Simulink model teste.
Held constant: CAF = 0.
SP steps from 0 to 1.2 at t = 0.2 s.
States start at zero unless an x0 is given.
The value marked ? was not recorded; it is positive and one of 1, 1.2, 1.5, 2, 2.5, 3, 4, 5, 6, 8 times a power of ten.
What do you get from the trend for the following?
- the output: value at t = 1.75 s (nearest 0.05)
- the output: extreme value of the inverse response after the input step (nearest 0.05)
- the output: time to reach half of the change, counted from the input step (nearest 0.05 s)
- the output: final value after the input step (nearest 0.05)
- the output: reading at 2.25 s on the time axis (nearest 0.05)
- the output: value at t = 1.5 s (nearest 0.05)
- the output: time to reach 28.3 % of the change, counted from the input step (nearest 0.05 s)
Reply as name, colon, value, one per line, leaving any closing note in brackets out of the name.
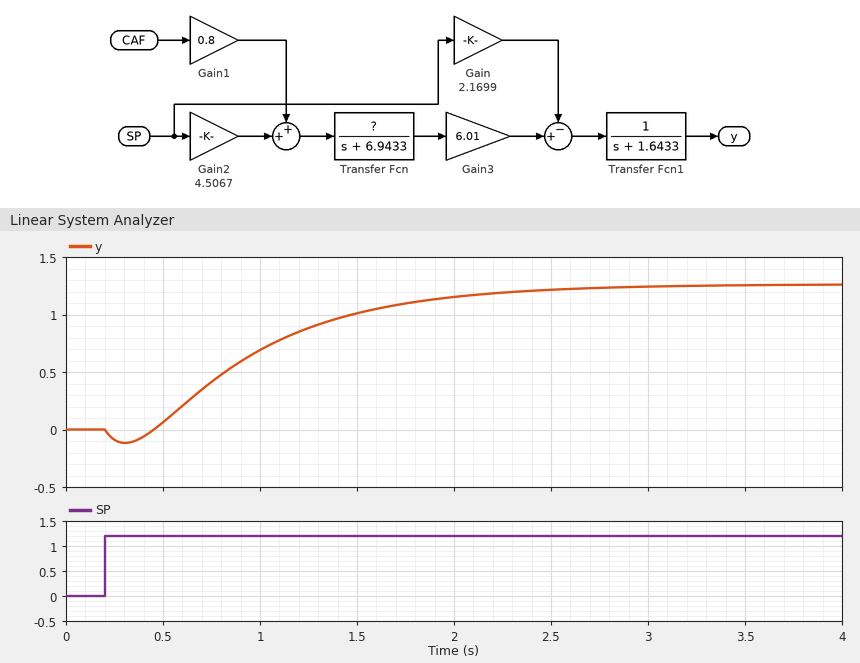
the output: value at t = 1.75 s: 1.10
the output: extreme value of the inverse response after the input step: -0.10
the output: time to reach half of the change, counted from the input step: 0.75 s
the output: final value after the input step: 1.25
the output: reading at 2.25 s on the time axis: 1.20
the output: value at t = 1.5 s: 1.00
the output: time to reach 28.3 % of the change, counted from the input step: 0.50 s
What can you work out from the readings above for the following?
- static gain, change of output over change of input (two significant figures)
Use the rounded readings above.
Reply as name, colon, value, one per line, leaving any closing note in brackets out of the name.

static gain, change of output over change of input: 1.0
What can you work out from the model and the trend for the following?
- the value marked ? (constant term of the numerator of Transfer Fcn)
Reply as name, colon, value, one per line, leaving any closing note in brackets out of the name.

the value marked ?: 1
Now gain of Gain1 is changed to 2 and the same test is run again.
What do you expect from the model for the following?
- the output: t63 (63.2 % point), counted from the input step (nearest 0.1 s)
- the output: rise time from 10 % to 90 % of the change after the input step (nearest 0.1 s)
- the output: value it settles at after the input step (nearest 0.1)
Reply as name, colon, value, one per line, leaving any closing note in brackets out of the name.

the output: t63 (63.2 % point), counted from the input step: 0.9 s
the output: rise time from 10 % to 90 % of the change after the input step: 1.4 s
the output: value it settles at after the input step: 1.3
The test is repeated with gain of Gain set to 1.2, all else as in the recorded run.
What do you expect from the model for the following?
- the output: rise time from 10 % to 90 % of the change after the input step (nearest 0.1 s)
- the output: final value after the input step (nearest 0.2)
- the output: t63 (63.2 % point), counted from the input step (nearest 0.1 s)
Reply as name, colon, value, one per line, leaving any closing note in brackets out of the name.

the output: rise time from 10 % to 90 % of the change after the input step: 1.4 s
the output: final value after the input step: 2.0
the output: t63 (63.2 % point), counted from the input step: 0.8 s
